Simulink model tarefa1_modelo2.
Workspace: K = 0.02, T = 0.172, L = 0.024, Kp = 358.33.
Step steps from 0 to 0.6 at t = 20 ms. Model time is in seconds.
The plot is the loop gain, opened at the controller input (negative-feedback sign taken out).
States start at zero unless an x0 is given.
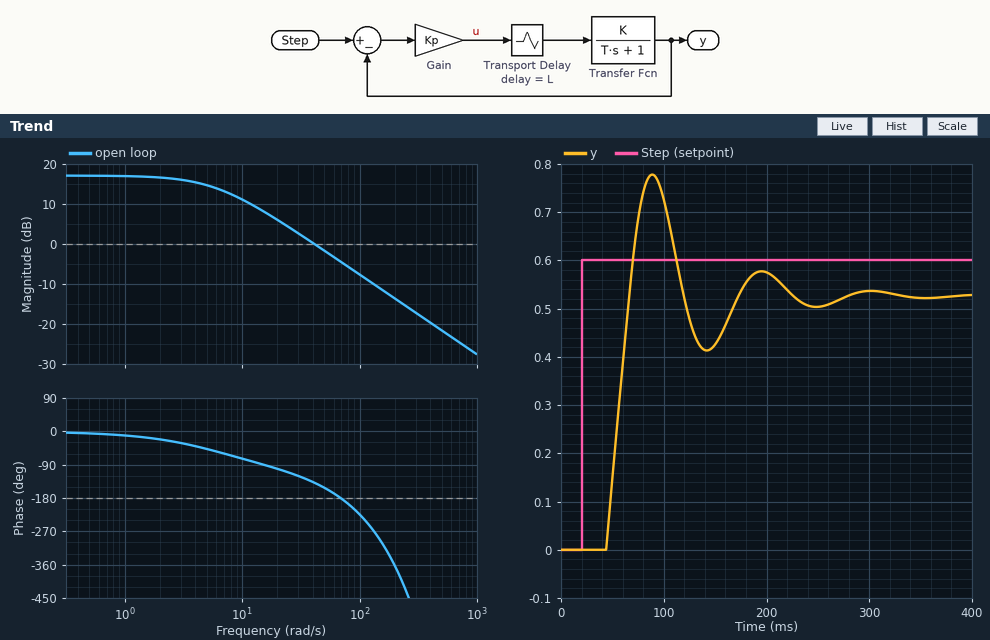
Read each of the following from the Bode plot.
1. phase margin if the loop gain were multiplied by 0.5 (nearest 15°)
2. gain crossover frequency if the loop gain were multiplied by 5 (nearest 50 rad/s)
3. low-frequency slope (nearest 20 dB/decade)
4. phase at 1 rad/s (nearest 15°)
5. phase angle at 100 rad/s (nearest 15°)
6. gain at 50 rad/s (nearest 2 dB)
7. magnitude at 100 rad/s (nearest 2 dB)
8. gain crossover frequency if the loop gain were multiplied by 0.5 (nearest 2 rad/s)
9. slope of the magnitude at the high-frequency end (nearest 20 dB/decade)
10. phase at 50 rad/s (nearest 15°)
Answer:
75°
200 rad/s
0 dB/decade
-15°
-225°
-2 dB
-8 dB
20 rad/s
-20 dB/decade
-150°
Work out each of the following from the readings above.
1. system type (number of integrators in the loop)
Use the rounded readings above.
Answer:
0
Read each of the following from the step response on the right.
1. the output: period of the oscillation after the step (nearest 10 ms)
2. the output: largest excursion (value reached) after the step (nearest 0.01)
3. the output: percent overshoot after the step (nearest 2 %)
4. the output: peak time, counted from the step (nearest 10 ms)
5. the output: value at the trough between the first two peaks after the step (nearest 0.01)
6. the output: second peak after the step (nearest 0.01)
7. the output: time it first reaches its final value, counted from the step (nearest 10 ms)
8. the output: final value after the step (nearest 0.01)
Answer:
110 ms
0.78
48 %
70 ms
0.41
0.58
50 ms
0.53
